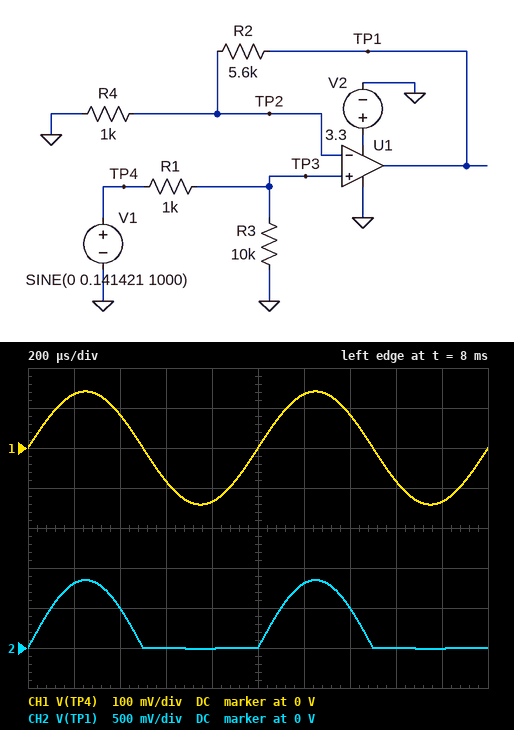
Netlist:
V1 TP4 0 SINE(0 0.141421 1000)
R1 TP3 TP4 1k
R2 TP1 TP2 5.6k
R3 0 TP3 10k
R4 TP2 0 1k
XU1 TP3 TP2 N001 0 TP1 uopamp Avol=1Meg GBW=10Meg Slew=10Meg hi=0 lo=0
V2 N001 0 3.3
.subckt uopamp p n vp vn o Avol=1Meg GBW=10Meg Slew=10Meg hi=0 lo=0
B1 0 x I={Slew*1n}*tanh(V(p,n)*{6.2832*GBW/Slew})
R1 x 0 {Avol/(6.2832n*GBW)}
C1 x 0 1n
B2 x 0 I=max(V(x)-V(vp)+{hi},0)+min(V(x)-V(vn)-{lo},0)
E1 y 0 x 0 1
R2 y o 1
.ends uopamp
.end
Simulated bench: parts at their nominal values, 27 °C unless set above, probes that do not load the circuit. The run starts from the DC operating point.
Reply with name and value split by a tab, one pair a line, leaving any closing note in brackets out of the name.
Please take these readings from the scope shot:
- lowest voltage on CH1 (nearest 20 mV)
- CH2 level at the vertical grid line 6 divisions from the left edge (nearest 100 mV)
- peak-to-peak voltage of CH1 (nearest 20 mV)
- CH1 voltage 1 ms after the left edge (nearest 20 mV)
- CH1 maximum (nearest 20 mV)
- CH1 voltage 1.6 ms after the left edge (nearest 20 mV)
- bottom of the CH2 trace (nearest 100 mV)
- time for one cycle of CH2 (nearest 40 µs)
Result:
lowest voltage on CH1	-140 mV
CH2 level at the vertical grid line 6 divisions from the left edge	800 mV
peak-to-peak voltage of CH1	280 mV
CH1 voltage 1 ms after the left edge	0 V
CH1 maximum	140 mV
CH1 voltage 1.6 ms after the left edge	-80 mV
bottom of the CH2 trace	0 V
time for one cycle of CH2	1.00 ms
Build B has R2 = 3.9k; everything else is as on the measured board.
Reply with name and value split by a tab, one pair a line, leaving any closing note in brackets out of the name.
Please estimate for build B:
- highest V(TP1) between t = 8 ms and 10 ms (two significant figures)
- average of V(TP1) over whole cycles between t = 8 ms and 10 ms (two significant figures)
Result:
highest V(TP1) between t = 8 ms and 10 ms	630 mV
average of V(TP1) over whole cycles between t = 8 ms and 10 ms	200 mV
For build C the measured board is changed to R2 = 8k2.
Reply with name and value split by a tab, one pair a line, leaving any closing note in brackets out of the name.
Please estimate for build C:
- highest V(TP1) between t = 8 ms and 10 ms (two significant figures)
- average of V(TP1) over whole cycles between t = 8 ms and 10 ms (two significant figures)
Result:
highest V(TP1) between t = 8 ms and 10 ms	1.2 V
average of V(TP1) over whole cycles between t = 8 ms and 10 ms	370 mV
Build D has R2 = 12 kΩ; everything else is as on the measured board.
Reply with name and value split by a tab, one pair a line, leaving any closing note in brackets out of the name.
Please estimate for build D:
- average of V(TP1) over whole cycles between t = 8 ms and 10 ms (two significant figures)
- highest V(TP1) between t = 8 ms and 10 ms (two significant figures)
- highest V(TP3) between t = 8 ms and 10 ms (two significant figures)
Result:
average of V(TP1) over whole cycles between t = 8 ms and 10 ms	530 mV
highest V(TP1) between t = 8 ms and 10 ms	1.7 V
highest V(TP3) between t = 8 ms and 10 ms	130 mV
